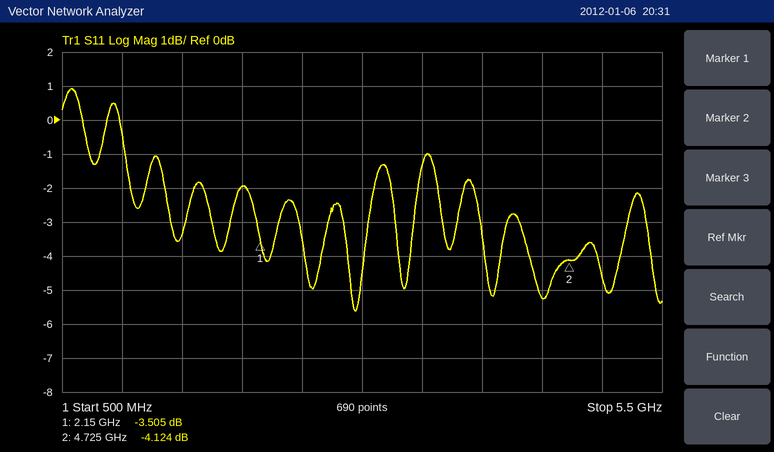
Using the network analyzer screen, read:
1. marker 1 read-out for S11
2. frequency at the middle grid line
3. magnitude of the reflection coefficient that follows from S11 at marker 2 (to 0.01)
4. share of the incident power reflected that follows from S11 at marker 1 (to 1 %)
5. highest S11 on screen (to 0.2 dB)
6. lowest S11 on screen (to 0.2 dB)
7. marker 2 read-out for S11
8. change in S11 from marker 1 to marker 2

-3.505 dB
3 GHz
0.62
45 %
1.0 dB
-5.6 dB
-4.124 dB
-0.619 dB
